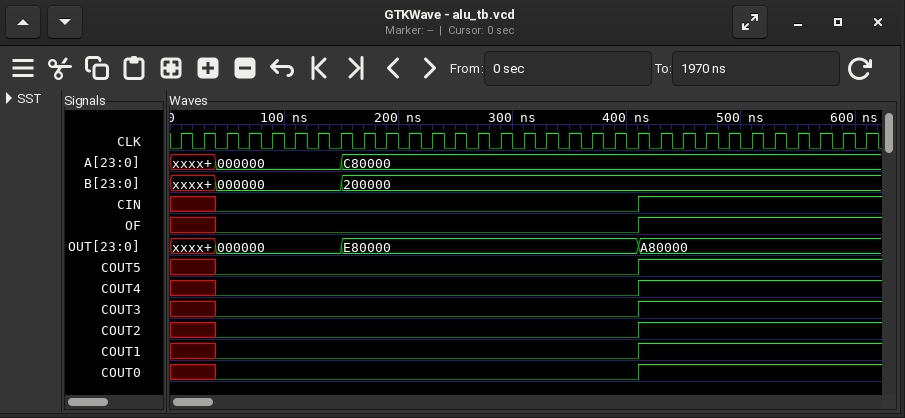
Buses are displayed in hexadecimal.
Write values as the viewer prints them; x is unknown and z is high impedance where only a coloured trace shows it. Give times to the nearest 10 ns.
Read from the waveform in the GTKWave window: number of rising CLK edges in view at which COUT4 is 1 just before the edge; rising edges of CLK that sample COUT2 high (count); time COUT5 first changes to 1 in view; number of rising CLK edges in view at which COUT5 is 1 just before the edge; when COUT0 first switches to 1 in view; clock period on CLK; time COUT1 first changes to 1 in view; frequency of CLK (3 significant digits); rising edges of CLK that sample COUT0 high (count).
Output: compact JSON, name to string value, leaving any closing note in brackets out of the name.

{"number of rising CLK edges in view at which COUT4 is 1 just before the edge": "10", "rising edges of CLK that sample COUT2 high": "10", "time COUT5 first changes to 1 in view": "410 ns", "number of rising CLK edges in view at which COUT5 is 1 just before the edge": "10", "when COUT0 first switches to 1 in view": "410 ns", "clock period on CLK": "20 ns", "time COUT1 first changes to 1 in view": "410 ns", "frequency of CLK": "50.0 MHz", "rising edges of CLK that sample COUT0 high": "10"}
